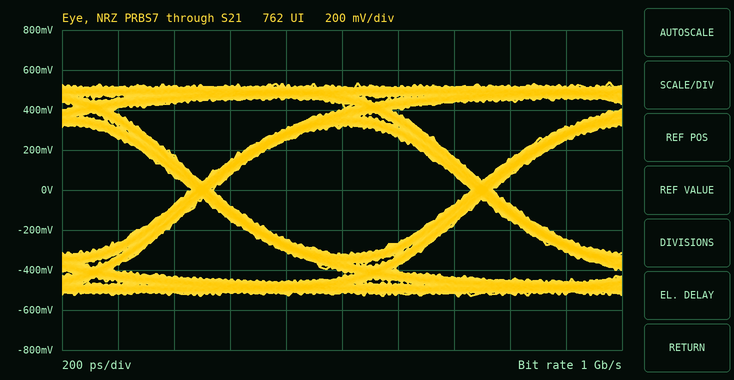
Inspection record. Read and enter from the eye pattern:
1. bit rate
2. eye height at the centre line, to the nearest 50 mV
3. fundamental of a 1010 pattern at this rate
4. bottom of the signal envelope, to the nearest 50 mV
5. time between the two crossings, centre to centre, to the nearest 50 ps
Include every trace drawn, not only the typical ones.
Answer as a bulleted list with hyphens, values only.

- 1 Gb/s
- 650 mV
- 500 MHz
- -550 mV
- 1.00 ns
